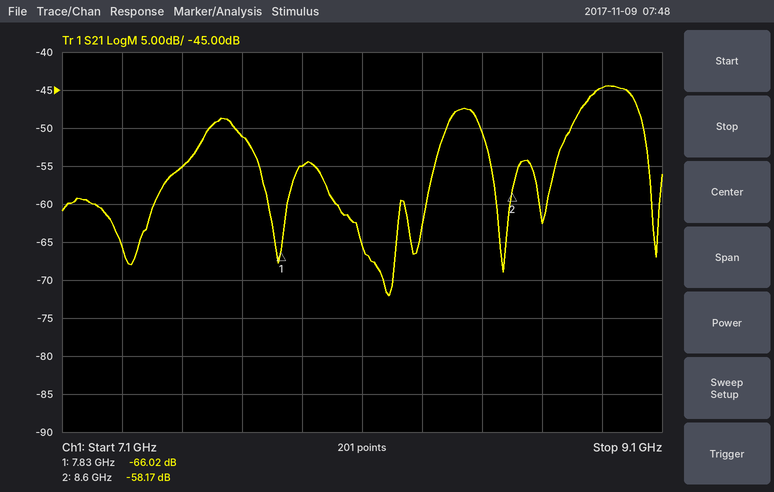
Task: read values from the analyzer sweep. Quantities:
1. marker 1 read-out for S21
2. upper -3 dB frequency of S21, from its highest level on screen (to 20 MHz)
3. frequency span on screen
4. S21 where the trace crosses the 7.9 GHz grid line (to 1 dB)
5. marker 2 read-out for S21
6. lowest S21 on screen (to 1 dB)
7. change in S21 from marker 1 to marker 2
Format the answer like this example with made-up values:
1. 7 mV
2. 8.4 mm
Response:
1. -66.02 dB
2. 9.02 GHz
3. 2 GHz
4. -55 dB
5. -58.17 dB
6. -72 dB
7. 7.85 dB
